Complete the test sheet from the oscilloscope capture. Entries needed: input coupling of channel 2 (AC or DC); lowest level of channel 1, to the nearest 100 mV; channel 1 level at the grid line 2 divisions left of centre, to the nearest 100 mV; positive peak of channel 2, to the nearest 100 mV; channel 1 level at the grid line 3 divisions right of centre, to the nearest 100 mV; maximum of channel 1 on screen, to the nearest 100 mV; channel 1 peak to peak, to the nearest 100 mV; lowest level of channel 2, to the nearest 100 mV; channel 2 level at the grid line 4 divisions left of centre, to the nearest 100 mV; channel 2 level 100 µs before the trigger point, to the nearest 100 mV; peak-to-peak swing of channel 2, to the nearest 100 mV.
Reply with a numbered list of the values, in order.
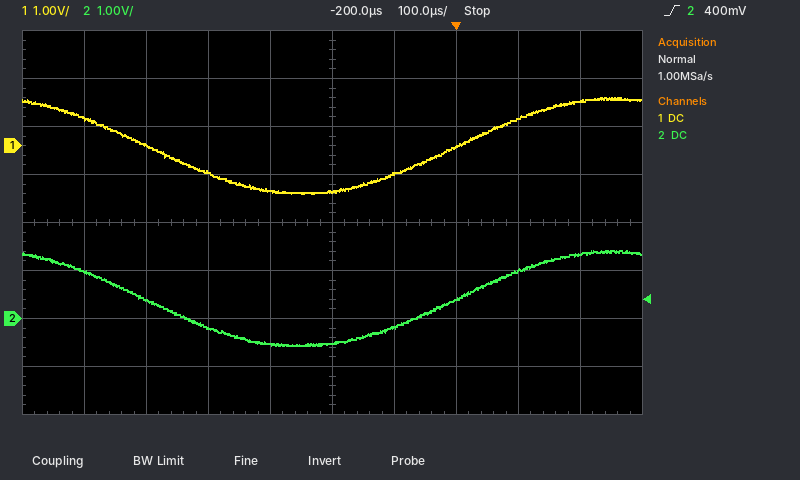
1. DC
2. -1.0 V
3. -600 mV
4. 1.4 V
5. 600 mV
6. 1.0 V
7. 2.0 V
8. -600 mV
9. 1.0 V
10. -200 mV
11. 2.0 V
